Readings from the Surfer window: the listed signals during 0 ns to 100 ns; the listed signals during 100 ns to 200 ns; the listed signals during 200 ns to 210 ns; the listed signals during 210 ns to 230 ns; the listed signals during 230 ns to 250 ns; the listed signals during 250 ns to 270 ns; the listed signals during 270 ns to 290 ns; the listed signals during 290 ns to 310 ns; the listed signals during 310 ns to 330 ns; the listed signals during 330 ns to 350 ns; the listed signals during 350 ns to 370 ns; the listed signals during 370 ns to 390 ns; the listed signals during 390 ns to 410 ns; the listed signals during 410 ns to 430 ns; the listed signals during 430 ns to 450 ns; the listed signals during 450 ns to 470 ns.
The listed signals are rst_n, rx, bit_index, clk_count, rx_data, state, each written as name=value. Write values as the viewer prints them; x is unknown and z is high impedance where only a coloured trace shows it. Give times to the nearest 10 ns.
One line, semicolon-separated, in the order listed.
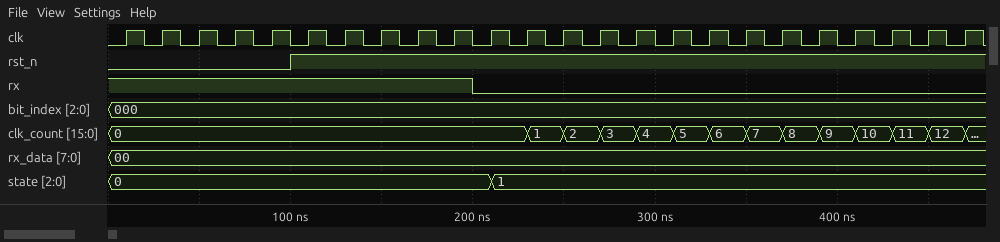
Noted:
rst_n=0, rx=1, bit_index=000, clk_count=0, rx_data=00, state=0; rst_n=1, rx=1, bit_index=000, clk_count=0, rx_data=00, state=0; rst_n=1, rx=0, bit_index=000, clk_count=0, rx_data=00, state=0; rst_n=1, rx=0, bit_index=000, clk_count=0, rx_data=00, state=1; rst_n=1, rx=0, bit_index=000, clk_count=1, rx_data=00, state=1; rst_n=1, rx=0, bit_index=000, clk_count=2, rx_data=00, state=1; rst_n=1, rx=0, bit_index=000, clk_count=3, rx_data=00, state=1; rst_n=1, rx=0, bit_index=000, clk_count=4, rx_data=00, state=1; rst_n=1, rx=0, bit_index=000, clk_count=5, rx_data=00, state=1; rst_n=1, rx=0, bit_index=000, clk_count=6, rx_data=00, state=1; rst_n=1, rx=0, bit_index=000, clk_count=7, rx_data=00, state=1; rst_n=1, rx=0, bit_index=000, clk_count=8, rx_data=00, state=1; rst_n=1, rx=0, bit_index=000, clk_count=9, rx_data=00, state=1; rst_n=1, rx=0, bit_index=000, clk_count=10, rx_data=00, state=1; rst_n=1, rx=0, bit_index=000, clk_count=11, rx_data=00, state=1; rst_n=1, rx=0, bit_index=000, clk_count=12, rx_data=00, state=1
